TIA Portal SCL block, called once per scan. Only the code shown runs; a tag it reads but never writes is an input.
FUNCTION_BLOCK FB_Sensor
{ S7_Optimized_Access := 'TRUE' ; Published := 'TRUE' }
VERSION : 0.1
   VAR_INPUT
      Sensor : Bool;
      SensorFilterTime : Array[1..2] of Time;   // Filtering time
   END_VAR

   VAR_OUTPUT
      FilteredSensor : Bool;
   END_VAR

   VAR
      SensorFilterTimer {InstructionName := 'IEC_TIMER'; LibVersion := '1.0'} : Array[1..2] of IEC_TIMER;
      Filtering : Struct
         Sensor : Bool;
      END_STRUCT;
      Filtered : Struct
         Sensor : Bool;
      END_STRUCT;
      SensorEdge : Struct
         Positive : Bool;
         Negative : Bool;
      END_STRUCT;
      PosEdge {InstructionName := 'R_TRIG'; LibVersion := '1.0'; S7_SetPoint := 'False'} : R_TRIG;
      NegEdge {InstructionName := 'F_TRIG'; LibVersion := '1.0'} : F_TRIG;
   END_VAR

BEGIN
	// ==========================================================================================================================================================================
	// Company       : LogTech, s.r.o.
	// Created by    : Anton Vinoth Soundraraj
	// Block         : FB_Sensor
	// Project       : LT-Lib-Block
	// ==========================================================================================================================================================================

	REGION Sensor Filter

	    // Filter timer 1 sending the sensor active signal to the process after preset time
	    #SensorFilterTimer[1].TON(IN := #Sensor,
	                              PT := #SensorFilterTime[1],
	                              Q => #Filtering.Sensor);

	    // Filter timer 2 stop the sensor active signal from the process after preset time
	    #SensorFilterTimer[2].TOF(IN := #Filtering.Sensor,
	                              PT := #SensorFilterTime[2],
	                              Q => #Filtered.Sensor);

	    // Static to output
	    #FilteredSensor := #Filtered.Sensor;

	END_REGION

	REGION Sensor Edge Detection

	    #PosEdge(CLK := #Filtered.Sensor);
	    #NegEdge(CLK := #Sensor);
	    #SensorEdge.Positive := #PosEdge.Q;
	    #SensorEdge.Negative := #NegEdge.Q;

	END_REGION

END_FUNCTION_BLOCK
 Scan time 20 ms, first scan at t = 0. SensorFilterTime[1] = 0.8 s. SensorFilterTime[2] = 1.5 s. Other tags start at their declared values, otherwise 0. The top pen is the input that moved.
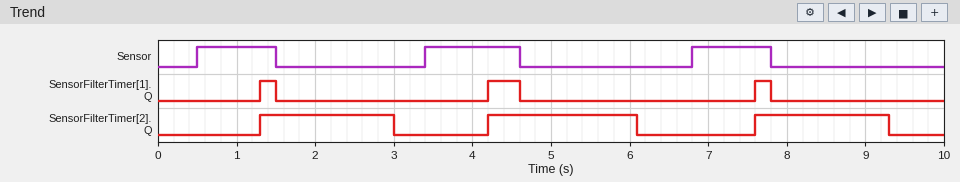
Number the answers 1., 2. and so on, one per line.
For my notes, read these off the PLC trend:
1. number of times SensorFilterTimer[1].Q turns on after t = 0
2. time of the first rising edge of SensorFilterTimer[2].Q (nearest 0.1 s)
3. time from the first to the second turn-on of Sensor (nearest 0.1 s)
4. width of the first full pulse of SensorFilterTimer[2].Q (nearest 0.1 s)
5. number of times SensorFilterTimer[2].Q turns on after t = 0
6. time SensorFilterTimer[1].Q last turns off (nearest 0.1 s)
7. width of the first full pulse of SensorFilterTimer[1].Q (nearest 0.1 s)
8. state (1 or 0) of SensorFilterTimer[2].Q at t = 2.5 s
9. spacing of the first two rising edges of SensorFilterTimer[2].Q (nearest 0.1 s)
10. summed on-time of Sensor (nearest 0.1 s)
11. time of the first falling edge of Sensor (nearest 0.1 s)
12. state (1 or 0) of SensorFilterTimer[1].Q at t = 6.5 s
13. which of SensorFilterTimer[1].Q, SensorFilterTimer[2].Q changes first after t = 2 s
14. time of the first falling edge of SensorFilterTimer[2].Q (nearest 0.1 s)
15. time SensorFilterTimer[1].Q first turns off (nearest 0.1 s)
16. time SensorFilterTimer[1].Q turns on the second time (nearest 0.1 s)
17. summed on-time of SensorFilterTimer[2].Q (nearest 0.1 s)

1. 3
2. 1.3 s
3. 2.9 s
4. 1.7 s
5. 3
6. 7.8 s
7. 0.2 s
8. 1
9. 2.9 s
10. 3.2 s
11. 1.5 s
12. 0
13. SensorFilterTimer[2].Q
14. 3.0 s
15. 1.5 s
16. 4.2 s
17. 5.3 s
